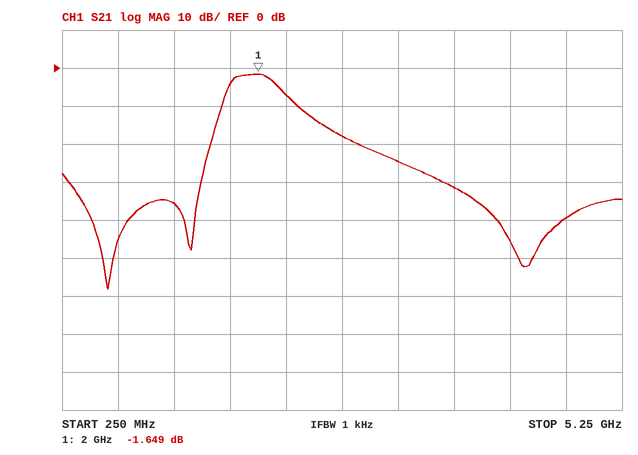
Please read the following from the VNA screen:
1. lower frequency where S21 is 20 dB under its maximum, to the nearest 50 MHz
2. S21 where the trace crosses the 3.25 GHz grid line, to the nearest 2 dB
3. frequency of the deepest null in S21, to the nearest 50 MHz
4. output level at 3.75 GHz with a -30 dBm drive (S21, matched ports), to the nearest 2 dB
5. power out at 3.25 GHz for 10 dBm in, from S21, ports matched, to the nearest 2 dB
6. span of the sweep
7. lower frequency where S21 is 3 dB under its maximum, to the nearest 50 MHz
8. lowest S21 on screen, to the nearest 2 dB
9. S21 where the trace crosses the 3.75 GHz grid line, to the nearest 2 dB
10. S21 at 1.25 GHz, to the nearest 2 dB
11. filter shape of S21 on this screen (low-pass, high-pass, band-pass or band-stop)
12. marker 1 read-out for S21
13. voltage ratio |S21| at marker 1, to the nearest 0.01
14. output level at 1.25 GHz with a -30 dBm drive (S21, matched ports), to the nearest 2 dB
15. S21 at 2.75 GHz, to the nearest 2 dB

1.55 GHz
-24 dB
650 MHz
-62 dBm
-14 dBm
5 GHz
1.75 GHz
-58 dB
-32 dB
-36 dB
band-pass
-1.649 dB
0.83
-66 dBm
-18 dB
